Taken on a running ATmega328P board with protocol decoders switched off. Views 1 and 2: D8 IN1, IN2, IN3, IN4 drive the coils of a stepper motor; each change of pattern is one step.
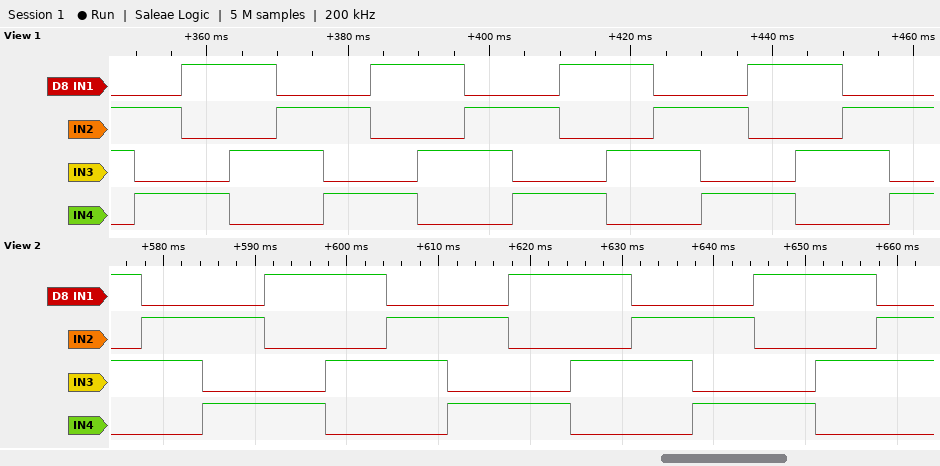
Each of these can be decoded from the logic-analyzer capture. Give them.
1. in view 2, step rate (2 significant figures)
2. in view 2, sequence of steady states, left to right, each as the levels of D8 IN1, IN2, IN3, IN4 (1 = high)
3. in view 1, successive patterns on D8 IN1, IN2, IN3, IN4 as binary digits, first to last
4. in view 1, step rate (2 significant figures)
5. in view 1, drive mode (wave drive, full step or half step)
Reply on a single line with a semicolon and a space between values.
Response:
150 steps/s; 1010 0110 0101 1001 1010 0110 0101 1001 1010 0110 0101 1001 1010 0110; 0110 0101 1001 1010 0110 0101 1001 1010 0110 0101 1001 1010 0110 0101 1001 1010 0110 0101; 150 steps/s; full step
